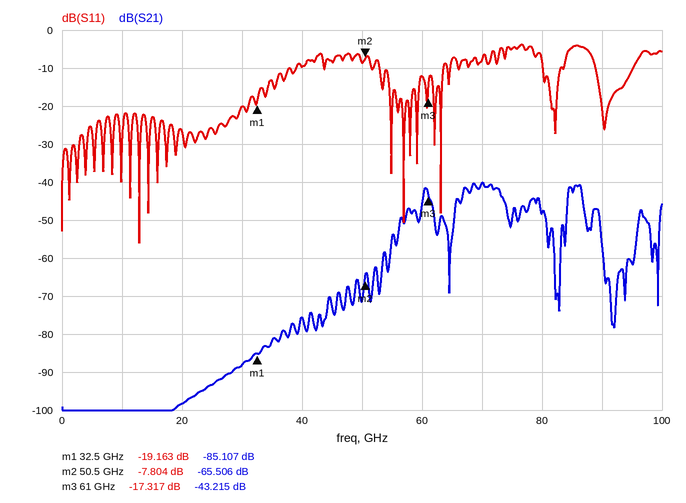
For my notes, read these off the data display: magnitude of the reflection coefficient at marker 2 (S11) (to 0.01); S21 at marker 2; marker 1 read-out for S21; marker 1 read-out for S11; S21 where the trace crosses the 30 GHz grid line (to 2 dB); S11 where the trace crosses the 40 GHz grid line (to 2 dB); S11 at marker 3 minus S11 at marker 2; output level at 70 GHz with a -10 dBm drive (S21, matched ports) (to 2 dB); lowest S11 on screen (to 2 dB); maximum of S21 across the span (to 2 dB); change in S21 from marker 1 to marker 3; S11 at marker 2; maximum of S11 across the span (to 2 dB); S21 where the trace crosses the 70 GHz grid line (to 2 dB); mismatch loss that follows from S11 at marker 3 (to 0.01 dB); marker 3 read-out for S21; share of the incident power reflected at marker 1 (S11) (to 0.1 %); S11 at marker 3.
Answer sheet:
0.41
-65.506 dB
-85.107 dB
-19.163 dB
-88 dB
-10 dB
-9.513 dB
-50 dBm
-56 dB
-40 dB
41.892 dB
-7.804 dB
-4 dB
-40 dB
0.08 dB
-43.215 dB
1.2 %
-17.317 dB
